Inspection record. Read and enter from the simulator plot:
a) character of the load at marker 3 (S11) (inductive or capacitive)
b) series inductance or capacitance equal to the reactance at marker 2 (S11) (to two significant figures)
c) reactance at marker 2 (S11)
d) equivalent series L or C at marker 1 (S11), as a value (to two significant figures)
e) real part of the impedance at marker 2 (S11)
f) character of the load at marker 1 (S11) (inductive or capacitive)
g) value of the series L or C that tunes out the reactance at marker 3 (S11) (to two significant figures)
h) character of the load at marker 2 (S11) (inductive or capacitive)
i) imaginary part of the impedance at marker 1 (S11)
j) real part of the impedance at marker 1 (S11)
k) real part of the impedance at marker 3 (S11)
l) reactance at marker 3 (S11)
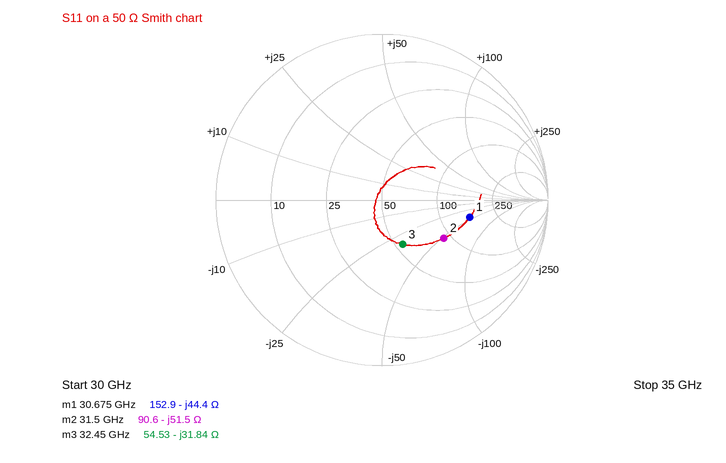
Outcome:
capacitive
98 fF
-51.5 Ω
120 fF
90.6 Ω
capacitive
160 pH
capacitive
-44.4 Ω
152.9 Ω
54.53 Ω
-31.84 Ω
